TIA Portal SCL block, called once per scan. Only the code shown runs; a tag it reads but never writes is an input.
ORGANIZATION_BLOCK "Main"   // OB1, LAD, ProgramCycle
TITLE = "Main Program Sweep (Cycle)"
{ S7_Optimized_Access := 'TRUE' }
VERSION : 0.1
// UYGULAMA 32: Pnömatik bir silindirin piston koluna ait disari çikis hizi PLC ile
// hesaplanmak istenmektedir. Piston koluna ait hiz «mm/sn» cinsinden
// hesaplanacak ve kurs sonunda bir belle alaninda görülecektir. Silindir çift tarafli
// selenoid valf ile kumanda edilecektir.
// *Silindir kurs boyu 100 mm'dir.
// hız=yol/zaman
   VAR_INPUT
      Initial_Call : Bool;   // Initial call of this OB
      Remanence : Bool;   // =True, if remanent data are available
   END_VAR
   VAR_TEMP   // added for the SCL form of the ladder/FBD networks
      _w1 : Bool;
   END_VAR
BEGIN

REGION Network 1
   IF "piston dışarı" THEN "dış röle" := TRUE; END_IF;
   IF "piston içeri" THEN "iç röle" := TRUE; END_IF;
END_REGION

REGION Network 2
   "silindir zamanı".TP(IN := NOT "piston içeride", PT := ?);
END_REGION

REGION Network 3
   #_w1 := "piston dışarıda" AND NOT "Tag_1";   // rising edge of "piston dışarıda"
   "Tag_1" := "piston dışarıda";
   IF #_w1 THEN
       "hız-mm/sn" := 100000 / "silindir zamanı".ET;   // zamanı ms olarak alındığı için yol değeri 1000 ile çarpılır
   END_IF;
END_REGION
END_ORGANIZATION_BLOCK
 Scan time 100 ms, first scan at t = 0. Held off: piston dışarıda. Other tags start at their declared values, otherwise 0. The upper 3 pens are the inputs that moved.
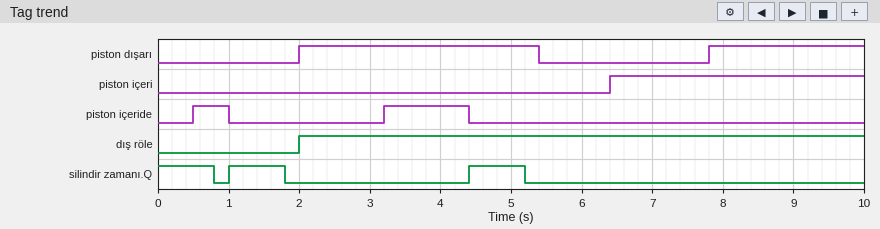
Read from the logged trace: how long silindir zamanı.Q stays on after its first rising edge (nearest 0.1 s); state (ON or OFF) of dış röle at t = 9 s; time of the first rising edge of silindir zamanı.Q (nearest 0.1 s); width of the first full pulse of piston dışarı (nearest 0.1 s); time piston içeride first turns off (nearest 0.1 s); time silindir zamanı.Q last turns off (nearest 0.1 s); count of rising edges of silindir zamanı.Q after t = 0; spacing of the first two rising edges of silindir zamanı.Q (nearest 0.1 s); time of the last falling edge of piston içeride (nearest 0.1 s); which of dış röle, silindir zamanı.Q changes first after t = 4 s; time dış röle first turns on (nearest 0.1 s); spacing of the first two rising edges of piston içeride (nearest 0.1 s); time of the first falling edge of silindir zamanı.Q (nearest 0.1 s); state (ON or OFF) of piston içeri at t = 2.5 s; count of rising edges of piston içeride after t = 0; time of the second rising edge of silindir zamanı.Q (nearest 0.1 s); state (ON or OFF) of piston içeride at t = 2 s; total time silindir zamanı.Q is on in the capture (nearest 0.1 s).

0.8 s
ON
1.0 s
3.4 s
1.0 s
5.2 s
2
3.4 s
4.4 s
silindir zamanı.Q
2.0 s
2.7 s
0.8 s
OFF
2
4.4 s
OFF
2.4 s
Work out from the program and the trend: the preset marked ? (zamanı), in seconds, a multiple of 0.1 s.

0.8 s
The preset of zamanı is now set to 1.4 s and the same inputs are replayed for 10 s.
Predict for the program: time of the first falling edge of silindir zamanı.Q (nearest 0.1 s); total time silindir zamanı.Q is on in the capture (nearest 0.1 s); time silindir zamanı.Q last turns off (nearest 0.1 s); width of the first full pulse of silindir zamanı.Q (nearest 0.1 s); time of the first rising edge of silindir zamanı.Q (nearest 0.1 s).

1.4 s
2.8 s
5.8 s
1.4 s
4.4 s
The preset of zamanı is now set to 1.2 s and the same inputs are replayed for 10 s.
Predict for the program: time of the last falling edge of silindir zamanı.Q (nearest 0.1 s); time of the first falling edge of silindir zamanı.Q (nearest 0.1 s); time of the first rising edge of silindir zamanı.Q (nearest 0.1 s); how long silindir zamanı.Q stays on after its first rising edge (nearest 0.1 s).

5.6 s
1.2 s
4.4 s
1.2 s
